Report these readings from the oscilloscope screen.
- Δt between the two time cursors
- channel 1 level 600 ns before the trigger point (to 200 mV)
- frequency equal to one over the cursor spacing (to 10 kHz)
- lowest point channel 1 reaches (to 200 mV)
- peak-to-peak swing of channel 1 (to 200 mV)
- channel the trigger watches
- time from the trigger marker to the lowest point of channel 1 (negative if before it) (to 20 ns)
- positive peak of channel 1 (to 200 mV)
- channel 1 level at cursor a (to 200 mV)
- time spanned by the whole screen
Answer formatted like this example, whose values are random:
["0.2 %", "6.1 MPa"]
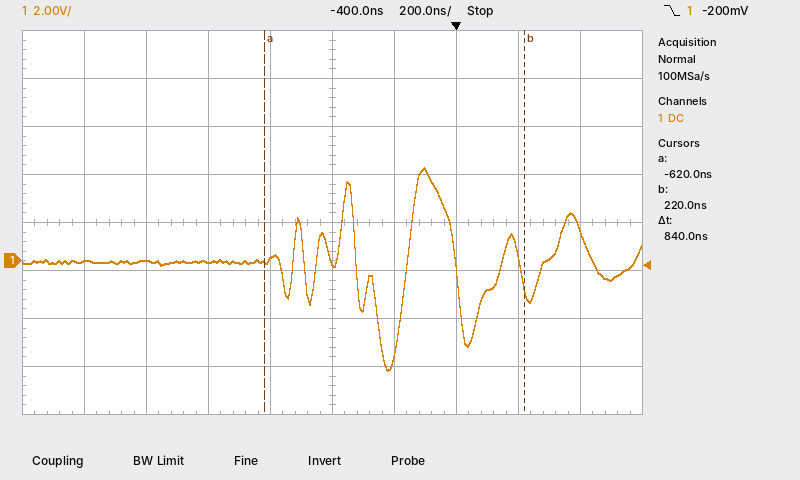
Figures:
["840 ns", "0.0 V", "1.19 MHz", "-4.6 V", "8.4 V", "channel 1", "-220 ns", "3.8 V", "0.0 V", "2 µs"]
